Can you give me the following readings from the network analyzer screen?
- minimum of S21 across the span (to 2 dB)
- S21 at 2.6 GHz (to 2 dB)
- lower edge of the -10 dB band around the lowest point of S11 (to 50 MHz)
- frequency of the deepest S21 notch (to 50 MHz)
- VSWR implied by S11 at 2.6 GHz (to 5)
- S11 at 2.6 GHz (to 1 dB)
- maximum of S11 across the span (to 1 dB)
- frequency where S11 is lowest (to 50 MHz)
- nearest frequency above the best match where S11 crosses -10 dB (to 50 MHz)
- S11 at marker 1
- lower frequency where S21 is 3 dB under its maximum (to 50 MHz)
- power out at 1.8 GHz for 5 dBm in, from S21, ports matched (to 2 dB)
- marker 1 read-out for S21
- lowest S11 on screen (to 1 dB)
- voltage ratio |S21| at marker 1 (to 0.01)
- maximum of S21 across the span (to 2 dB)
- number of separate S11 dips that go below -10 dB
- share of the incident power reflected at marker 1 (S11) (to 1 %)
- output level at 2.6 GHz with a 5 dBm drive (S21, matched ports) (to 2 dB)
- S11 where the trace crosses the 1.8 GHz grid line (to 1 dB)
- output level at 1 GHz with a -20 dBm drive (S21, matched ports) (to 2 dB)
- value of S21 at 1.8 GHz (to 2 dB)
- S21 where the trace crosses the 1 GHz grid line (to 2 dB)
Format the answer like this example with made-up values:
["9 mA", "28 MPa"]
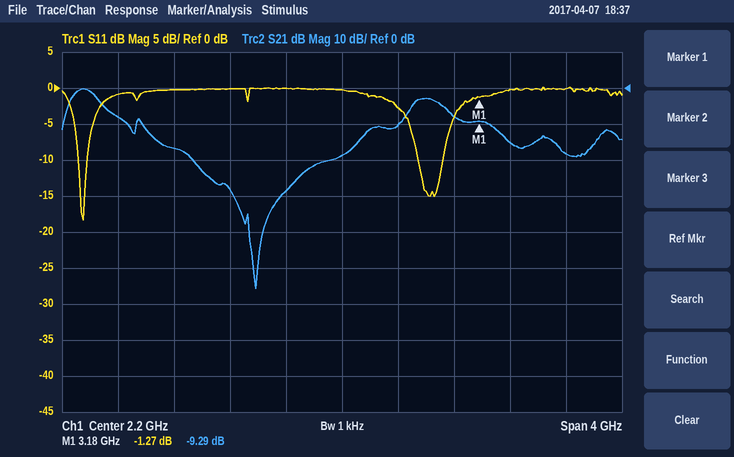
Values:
["-56 dB", "-10 dB", "300 MHz", "1.60 GHz", "5", "-3 dB", "0 dB", "350 MHz", "400 MHz", "-1.27 dB", "250 MHz", "-24 dBm", "-9.29 dB", "-18 dB", "0.34", "0 dB", "2", "75 %", "-6 dBm", "0 dB", "-36 dBm", "-28 dB", "-16 dB"]
